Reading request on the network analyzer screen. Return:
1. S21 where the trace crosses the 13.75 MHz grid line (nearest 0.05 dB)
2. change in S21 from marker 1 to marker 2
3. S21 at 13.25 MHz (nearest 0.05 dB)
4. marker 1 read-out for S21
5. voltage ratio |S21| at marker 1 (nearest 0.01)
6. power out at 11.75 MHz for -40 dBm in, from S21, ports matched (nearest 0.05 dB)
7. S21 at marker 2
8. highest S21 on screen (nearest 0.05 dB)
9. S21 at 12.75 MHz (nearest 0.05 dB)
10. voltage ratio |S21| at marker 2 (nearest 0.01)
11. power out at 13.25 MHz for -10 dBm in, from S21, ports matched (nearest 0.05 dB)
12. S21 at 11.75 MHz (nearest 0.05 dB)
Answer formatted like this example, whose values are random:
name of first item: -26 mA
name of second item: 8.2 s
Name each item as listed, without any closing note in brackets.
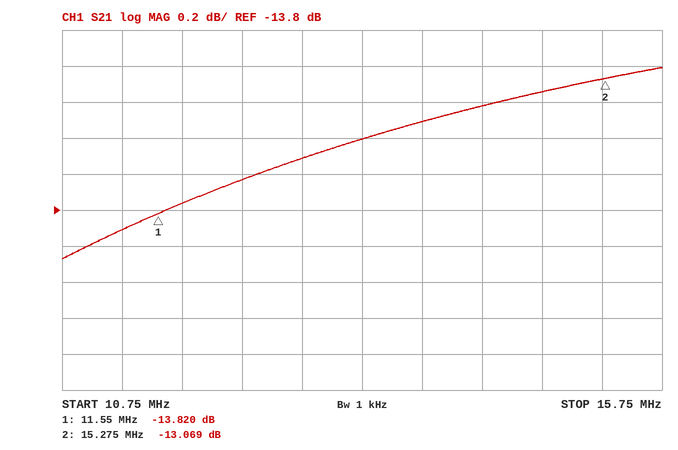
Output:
S21 where the trace crosses the 13.75 MHz grid line: -13.30 dB
change in S21 from marker 1 to marker 2: 0.751 dB
S21 at 13.25 MHz: -13.40 dB
marker 1 read-out for S21: -13.820 dB
voltage ratio |S21| at marker 1: 0.20
power out at 11.75 MHz for -40 dBm in, from S21, ports matched: -53.75 dBm
S21 at marker 2: -13.069 dB
highest S21 on screen: -13.00 dB
S21 at 12.75 MHz: -13.50 dB
voltage ratio |S21| at marker 2: 0.22
power out at 13.25 MHz for -10 dBm in, from S21, ports matched: -23.40 dBm
S21 at 11.75 MHz: -13.75 dB
